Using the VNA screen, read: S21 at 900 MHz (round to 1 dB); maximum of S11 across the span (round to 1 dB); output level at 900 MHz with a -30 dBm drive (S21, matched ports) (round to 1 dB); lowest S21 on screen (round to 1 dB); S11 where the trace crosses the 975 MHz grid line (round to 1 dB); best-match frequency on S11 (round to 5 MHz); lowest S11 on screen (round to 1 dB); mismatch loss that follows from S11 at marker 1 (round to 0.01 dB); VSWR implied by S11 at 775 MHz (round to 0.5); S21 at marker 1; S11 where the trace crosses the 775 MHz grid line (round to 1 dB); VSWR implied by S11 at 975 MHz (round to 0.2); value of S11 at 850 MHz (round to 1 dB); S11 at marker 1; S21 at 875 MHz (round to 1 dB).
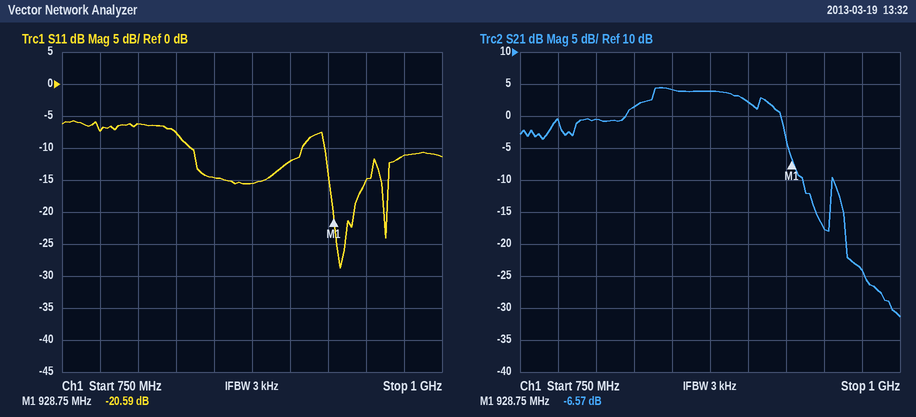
2 dB
-6 dB
-28 dBm
-31 dB
-11 dB
935 MHz
-29 dB
0.04 dB
2.5
-6.57 dB
-7 dB
1.8
-15 dB
-20.59 dB
4 dB
